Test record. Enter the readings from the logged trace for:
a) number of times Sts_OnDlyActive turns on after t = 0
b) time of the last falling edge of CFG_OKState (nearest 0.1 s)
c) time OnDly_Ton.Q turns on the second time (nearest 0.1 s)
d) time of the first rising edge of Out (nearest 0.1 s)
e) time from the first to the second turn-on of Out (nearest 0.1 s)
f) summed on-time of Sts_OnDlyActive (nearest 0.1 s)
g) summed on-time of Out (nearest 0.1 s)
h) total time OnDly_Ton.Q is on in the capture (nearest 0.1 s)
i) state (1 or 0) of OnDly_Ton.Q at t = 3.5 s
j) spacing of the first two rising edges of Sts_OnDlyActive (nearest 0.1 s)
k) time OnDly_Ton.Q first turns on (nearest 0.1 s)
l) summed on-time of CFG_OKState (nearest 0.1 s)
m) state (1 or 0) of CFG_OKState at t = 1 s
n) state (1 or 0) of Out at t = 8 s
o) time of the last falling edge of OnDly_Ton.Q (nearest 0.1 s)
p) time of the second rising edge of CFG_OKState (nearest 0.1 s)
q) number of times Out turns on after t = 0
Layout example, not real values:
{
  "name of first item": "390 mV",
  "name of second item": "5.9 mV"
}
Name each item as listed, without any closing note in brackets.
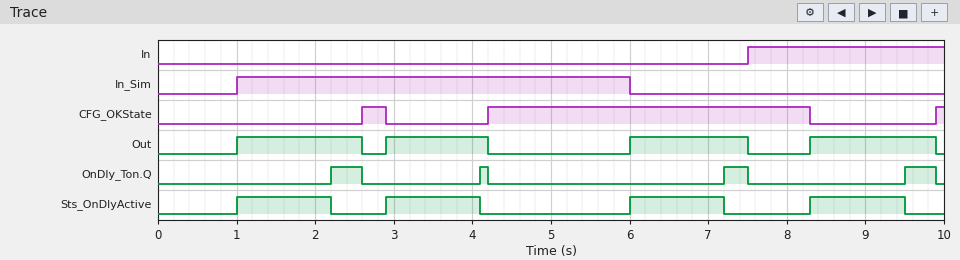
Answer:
{
  "number of times Sts_OnDlyActive turns on after t = 0": "4",
  "time of the last falling edge of CFG_OKState": "8.3 s",
  "time OnDly_Ton.Q turns on the second time": "4.1 s",
  "time of the first rising edge of Out": "1.0 s",
  "time from the first to the second turn-on of Out": "1.9 s",
  "summed on-time of Sts_OnDlyActive": "4.8 s",
  "summed on-time of Out": "6.0 s",
  "total time OnDly_Ton.Q is on in the capture": "1.2 s",
  "state (1 or 0) of OnDly_Ton.Q at t = 3.5 s": "0",
  "spacing of the first two rising edges of Sts_OnDlyActive": "1.9 s",
  "time OnDly_Ton.Q first turns on": "2.2 s",
  "summed on-time of CFG_OKState": "4.5 s",
  "state (1 or 0) of CFG_OKState at t = 1 s": "0",
  "state (1 or 0) of Out at t = 8 s": "0",
  "time of the last falling edge of OnDly_Ton.Q": "9.9 s",
  "time of the second rising edge of CFG_OKState": "4.2 s",
  "number of times Out turns on after t = 0": "4"
}
